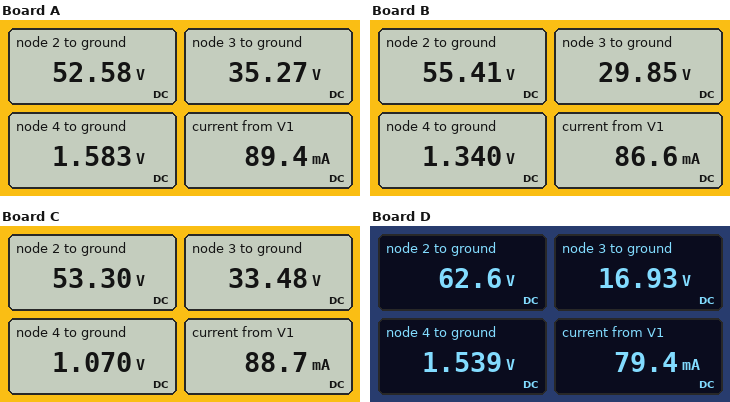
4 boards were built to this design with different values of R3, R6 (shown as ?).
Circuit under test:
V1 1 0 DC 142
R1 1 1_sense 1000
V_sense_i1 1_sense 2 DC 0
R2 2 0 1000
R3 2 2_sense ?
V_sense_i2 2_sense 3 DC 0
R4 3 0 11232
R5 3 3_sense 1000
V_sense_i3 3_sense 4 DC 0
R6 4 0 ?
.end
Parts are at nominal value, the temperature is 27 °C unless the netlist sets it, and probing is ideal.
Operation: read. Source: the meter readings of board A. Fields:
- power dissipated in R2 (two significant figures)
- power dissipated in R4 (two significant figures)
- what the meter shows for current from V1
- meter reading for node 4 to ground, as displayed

2.8 W
110 mW
89.4 mA
1.583 V
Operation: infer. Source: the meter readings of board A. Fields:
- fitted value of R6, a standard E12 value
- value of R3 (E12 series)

47 Ω
470 Ω
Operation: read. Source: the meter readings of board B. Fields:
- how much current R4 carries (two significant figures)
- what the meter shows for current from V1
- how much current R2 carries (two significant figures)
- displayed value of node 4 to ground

2.7 mA
86.6 mA
55 mA
1.340 V
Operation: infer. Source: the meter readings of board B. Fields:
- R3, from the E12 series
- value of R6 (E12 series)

820 Ω
47 Ω
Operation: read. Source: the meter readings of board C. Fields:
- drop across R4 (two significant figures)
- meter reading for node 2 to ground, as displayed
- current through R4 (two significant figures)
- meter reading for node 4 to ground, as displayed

33 V
53.30 V
3.0 mA
1.070 V
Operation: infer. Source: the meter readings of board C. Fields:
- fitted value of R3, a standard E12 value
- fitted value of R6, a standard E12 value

560 Ω
33 Ω
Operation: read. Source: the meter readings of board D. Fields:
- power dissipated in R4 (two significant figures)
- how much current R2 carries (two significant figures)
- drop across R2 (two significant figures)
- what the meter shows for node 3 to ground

26 mW
63 mA
63 V
16.93 V
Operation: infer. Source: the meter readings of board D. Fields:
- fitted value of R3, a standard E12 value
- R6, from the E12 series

2.7 kΩ
100 Ω
